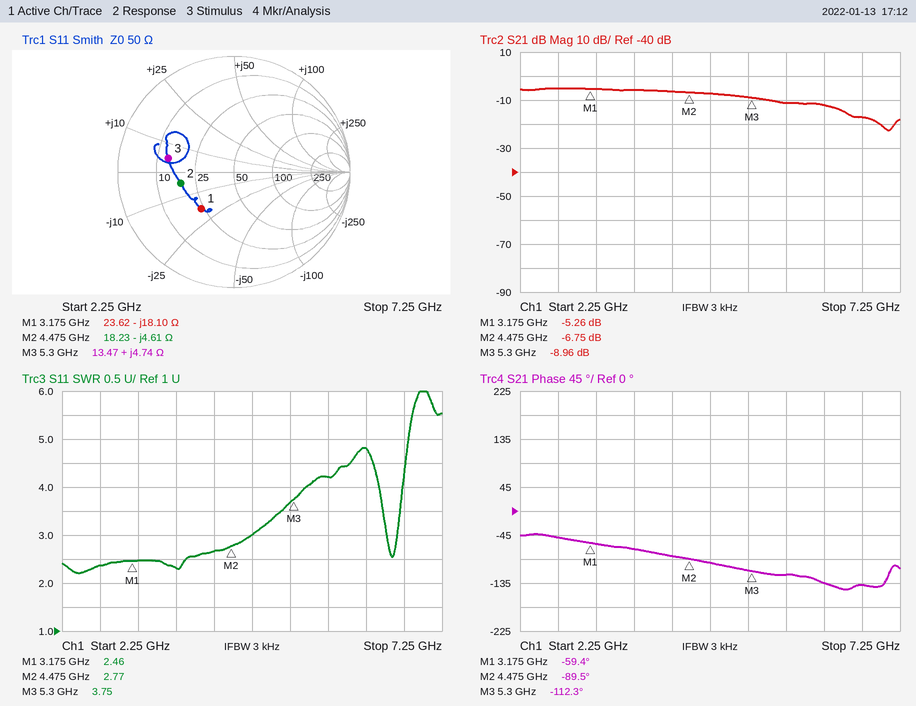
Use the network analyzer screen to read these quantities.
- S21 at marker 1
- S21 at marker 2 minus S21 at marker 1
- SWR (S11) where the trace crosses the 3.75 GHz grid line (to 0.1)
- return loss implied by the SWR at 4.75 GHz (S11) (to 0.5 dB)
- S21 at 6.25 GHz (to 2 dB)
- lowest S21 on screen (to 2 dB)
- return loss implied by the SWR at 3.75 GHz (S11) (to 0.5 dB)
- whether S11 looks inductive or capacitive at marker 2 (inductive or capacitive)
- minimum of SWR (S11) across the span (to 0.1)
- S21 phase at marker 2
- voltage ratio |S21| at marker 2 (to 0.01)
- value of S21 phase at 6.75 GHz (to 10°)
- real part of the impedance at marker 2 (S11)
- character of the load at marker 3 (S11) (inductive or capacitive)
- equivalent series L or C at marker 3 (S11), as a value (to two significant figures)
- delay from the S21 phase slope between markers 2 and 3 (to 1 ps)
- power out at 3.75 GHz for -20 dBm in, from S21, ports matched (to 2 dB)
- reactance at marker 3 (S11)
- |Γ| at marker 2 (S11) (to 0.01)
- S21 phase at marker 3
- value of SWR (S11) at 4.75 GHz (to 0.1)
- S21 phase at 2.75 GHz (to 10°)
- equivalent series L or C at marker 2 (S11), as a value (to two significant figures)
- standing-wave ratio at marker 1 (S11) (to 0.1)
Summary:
-5.26 dB
-1.49 dB
2.3
6.0 dB
-12 dB
-22 dB
8.0 dB
capacitive
2.2
-89.5°
0.46
-140°
18.23 Ω
inductive
140 pH
77 ps
-26 dBm
+4.74 Ω
0.47
-112.3°
3.0
-50°
7.7 pF
2.5
